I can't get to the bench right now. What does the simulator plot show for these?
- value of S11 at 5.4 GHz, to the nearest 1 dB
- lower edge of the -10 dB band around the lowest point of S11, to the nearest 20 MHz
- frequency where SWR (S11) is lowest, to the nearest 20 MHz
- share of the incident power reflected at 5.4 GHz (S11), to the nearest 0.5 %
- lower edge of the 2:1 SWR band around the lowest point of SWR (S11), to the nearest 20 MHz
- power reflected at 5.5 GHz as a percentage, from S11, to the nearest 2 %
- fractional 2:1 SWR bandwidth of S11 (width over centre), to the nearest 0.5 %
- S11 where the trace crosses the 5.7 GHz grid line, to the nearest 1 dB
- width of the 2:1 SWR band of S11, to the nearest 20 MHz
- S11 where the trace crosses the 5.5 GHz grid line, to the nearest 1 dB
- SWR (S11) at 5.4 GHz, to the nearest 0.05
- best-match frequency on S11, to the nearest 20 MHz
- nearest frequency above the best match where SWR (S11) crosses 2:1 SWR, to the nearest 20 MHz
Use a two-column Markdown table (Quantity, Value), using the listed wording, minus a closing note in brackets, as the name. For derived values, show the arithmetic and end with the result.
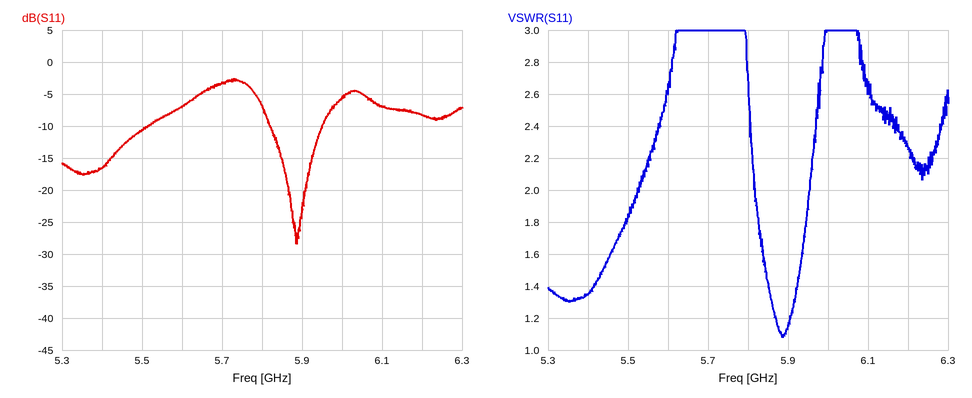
| Quantity | Value |
|---|---|
| value of S11 at 5.4 GHz, to the nearest 1 dB | -17 dB |
| lower edge of the -10 dB band around the lowest point of S11, to the nearest 20 MHz | 5.82 GHz |
| frequency where SWR (S11) is lowest, to the nearest 20 MHz | 5.88 GHz |
| share of the incident power reflected at 5.4 GHz (S11), to the nearest 0.5 % | 10^(-17/10) ≈ 2.0 % |
| lower edge of the 2:1 SWR band around the lowest point of SWR (S11), to the nearest 20 MHz | 5.82 GHz |
| power reflected at 5.5 GHz as a percentage, from S11, to the nearest 2 % | 10^(-11/10) ≈ 8 % |
| fractional 2:1 SWR bandwidth of S11 (width over centre), to the nearest 0.5 % | 140 MHz / 5.89 GHz ≈ 2.38 %, so 2.5 % to the nearest 0.5 % |
| S11 where the trace crosses the 5.7 GHz grid line, to the nearest 1 dB | -3 dB |
| width of the 2:1 SWR band of S11, to the nearest 20 MHz | 5.96 GHz − 5.82 GHz = 140 MHz |
| S11 where the trace crosses the 5.5 GHz grid line, to the nearest 1 dB | -11 dB |
| SWR (S11) at 5.4 GHz, to the nearest 0.05 | 1.35 |
| best-match frequency on S11, to the nearest 20 MHz | 5.88 GHz |
| nearest frequency above the best match where SWR (S11) crosses 2:1 SWR, to the nearest 20 MHz | 5.96 GHz |
